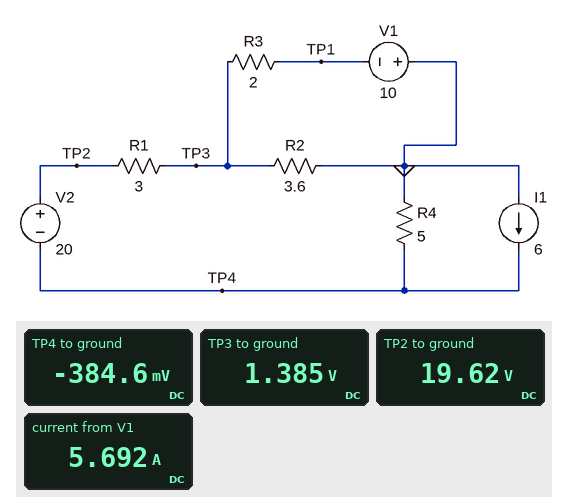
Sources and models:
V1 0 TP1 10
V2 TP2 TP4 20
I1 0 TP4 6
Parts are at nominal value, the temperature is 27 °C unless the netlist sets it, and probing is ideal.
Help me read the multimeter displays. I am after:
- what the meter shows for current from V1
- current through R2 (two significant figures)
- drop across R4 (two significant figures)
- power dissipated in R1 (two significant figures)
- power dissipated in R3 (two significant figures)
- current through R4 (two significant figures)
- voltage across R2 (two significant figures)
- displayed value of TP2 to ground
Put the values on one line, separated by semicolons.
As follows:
5.692 A; 380 mA; 380 mV; 110 W; 65 W; 77 mA; 1.4 V; 19.62 V
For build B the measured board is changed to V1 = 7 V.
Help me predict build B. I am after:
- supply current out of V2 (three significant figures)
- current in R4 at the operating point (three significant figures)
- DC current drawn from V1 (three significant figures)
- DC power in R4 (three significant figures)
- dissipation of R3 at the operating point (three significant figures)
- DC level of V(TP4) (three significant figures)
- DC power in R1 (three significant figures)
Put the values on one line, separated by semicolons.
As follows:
5.87 A; 131 mA; 5.02 A; 85.5 mW; 50.5 W; 654 mV; 103 W
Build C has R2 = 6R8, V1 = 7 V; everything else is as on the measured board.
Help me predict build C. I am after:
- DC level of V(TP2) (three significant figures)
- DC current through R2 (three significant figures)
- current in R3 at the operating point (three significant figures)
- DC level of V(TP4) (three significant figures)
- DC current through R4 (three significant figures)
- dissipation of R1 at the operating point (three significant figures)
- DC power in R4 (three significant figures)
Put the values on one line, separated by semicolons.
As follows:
21.0 V; 524 mA; 5.28 A; 976 mV; 195 mA; 101 W; 191 mW
